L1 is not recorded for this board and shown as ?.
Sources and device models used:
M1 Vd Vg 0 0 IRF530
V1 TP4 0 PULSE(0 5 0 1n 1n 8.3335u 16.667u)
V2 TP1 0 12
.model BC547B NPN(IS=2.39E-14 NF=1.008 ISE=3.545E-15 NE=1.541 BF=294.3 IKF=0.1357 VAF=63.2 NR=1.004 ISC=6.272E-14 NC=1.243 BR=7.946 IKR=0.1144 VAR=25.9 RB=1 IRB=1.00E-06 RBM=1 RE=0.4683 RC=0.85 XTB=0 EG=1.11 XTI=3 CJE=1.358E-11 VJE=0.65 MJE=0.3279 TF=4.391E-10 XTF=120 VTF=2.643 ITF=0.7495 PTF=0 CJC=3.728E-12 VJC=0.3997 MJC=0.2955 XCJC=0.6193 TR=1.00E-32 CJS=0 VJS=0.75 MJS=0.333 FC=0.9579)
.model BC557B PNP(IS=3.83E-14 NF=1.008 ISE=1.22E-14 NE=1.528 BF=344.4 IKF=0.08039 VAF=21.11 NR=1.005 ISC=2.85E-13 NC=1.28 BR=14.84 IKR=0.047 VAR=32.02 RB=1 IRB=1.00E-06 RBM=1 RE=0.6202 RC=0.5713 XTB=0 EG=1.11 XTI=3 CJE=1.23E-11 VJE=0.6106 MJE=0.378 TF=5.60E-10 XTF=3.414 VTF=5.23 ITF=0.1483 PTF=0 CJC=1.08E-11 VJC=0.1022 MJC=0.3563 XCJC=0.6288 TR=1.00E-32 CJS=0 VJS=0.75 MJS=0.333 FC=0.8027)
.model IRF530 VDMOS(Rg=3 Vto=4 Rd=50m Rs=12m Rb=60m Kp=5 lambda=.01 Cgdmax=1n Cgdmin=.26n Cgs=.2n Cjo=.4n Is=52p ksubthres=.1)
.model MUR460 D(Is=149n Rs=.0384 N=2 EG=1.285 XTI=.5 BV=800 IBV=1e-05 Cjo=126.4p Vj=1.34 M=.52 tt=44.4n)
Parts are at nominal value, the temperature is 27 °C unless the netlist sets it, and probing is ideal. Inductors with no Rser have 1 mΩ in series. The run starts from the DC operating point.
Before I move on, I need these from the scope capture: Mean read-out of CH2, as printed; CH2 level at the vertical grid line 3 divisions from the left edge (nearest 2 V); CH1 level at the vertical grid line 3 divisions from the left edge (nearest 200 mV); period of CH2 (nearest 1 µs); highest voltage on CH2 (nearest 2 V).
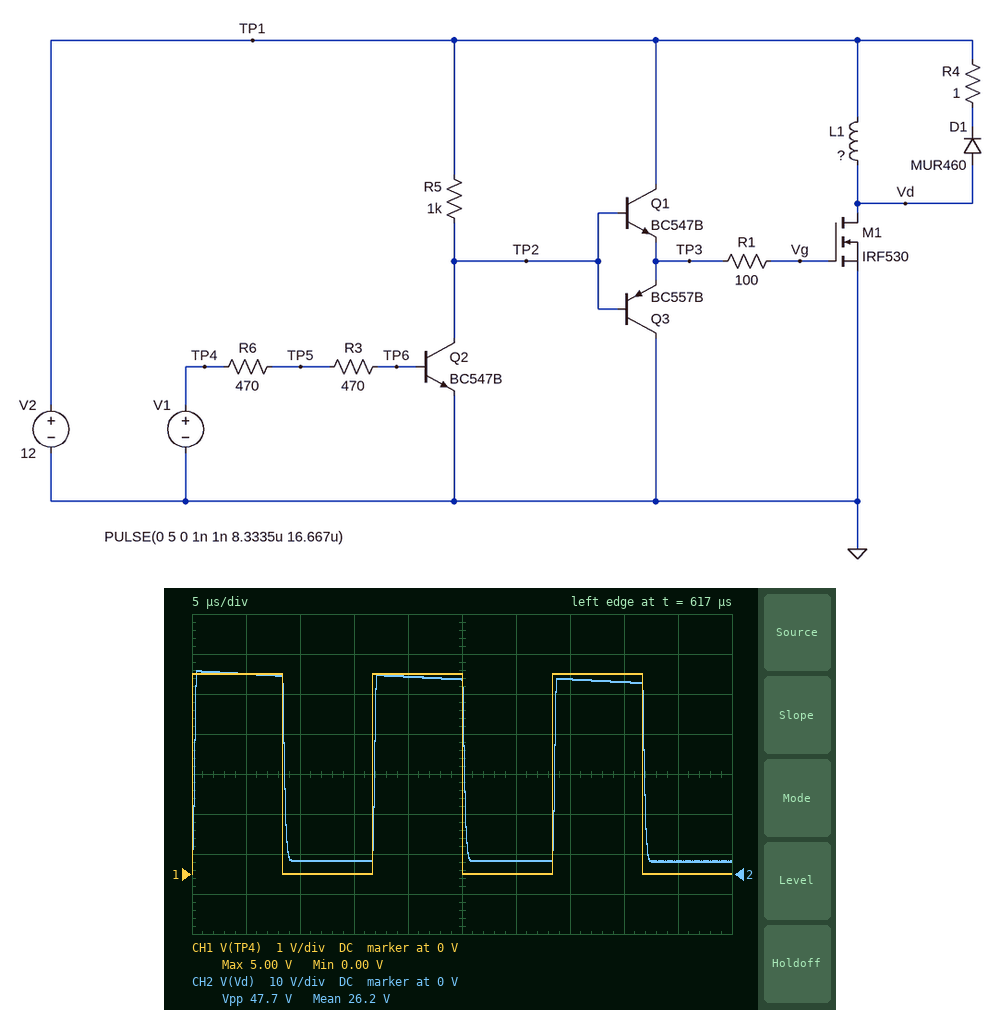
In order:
26.2 V
4 V
0 V
17 µs
50 V
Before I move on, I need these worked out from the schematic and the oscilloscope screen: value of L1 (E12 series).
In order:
270 µH
